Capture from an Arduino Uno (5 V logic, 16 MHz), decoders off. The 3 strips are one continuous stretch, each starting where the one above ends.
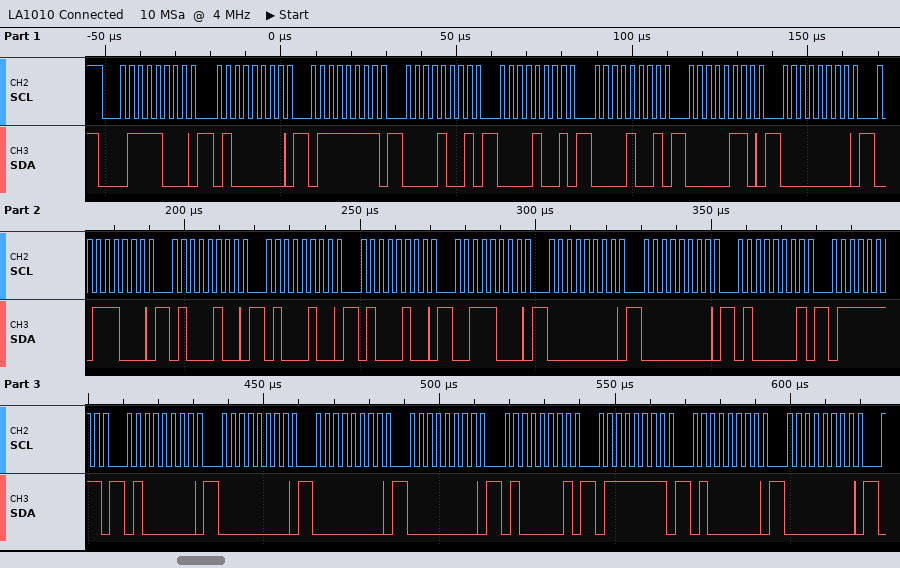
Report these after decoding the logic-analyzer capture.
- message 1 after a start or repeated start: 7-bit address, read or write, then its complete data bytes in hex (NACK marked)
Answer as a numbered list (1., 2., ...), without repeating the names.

1. 0x3C write: 40 7F 09 09 09 06 00 38 44 44 44 38 00 00 41 7F 40 00 00 00 41 7F 40 00
